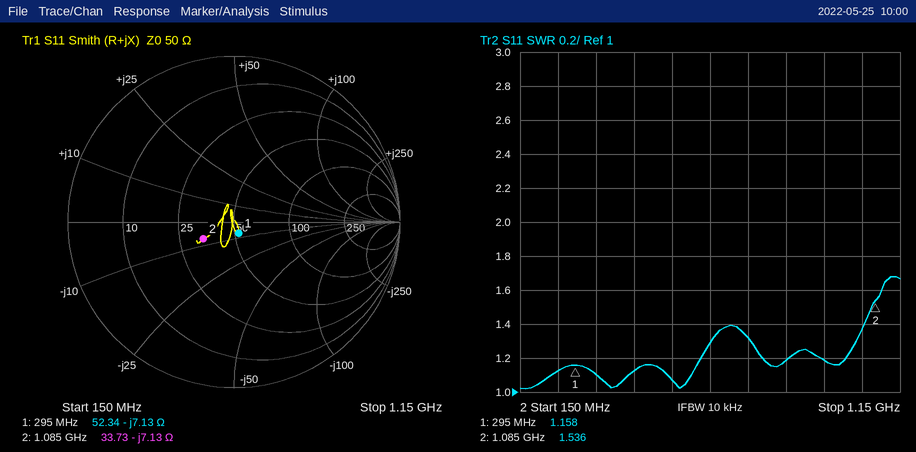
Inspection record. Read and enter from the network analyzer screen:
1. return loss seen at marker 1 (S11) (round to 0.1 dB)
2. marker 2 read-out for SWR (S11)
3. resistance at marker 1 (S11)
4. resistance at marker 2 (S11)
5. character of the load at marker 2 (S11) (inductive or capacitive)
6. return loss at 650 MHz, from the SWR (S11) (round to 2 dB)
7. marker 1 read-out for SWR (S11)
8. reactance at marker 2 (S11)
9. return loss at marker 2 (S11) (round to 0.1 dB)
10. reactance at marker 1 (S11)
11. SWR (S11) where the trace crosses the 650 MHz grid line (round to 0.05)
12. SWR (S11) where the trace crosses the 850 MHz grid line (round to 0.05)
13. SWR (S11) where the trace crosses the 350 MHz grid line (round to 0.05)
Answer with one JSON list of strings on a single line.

["22.7 dB", "1.536", "52.34 Ω", "33.73 Ω", "capacitive", "18 dB", "1.158", "-7.13 Ω", "13.5 dB", "-7.13 Ω", "1.30", "1.20", "1.10"]
